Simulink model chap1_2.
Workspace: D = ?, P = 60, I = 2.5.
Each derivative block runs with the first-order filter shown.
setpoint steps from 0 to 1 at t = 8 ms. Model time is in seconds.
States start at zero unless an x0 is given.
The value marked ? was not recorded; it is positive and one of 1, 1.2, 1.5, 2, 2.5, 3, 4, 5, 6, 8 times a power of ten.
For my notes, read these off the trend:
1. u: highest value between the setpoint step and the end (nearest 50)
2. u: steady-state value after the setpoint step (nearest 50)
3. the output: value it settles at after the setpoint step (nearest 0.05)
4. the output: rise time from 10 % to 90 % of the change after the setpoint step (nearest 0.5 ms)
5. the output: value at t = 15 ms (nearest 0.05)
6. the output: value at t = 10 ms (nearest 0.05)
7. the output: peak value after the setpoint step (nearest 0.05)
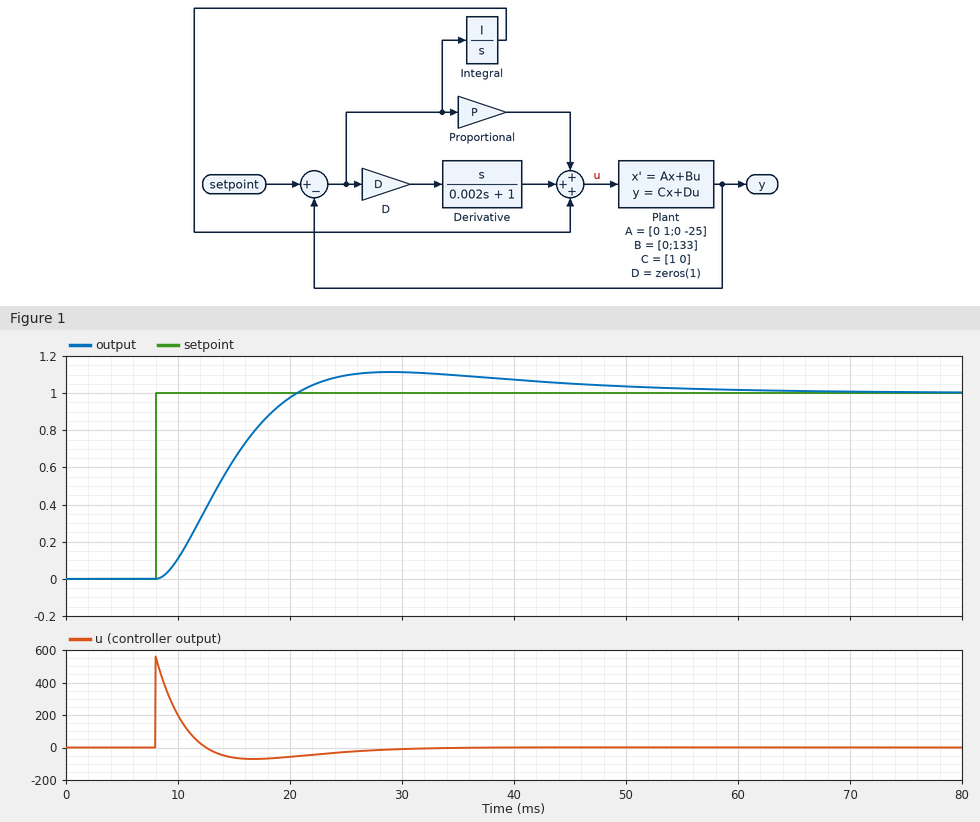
550
0
1.00
8.5 ms
0.65
0.10
1.10
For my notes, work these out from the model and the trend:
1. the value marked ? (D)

1
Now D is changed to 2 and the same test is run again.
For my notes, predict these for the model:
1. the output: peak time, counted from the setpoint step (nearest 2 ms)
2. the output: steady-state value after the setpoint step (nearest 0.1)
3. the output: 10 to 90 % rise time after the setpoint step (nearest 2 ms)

12 ms
1.0
6 ms
